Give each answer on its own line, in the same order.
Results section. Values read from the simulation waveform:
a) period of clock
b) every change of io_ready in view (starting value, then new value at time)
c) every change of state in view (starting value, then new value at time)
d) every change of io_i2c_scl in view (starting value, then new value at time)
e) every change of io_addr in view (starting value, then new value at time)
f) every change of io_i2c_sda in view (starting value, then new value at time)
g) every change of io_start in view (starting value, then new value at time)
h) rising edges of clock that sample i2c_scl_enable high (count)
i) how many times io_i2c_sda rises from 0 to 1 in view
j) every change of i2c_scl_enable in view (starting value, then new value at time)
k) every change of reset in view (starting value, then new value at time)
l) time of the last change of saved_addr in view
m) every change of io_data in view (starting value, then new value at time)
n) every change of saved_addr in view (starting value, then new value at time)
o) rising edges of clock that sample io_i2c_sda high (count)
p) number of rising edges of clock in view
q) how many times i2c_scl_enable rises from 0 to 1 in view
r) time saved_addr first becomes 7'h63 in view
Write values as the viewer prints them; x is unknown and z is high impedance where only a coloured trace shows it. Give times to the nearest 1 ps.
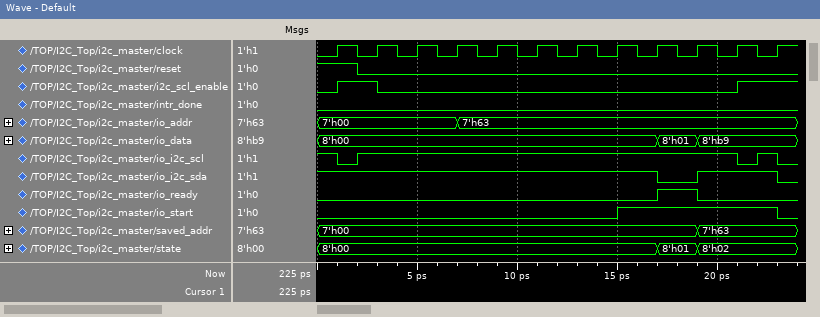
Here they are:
2 ps
0, 1 at 17 ps, 0 at 19 ps
8'h00, 8'h01 at 17 ps, 8'h02 at 19 ps
1, 0 at 1 ps, 1 at 2 ps, 0 at 21 ps, 1 at 22 ps, 0 at 23 ps
7'h00, 7'h63 at 7 ps
1, 0 at 17 ps, 1 at 19 ps, 0 at 23 ps
0, 1 at 15 ps, 0 at 23 ps
2
1
0, 1 at 1 ps, 0 at 3 ps, 1 at 21 ps
1, 0 at 2 ps
19 ps
8'h00, 8'h01 at 17 ps, 8'hb9 at 19 ps
7'h00, 7'h63 at 19 ps
11
12
2
19 ps
